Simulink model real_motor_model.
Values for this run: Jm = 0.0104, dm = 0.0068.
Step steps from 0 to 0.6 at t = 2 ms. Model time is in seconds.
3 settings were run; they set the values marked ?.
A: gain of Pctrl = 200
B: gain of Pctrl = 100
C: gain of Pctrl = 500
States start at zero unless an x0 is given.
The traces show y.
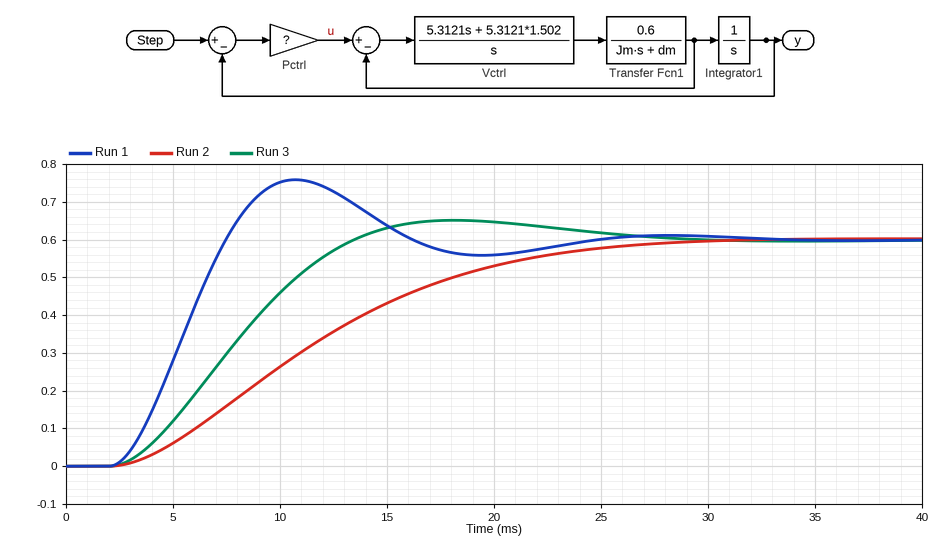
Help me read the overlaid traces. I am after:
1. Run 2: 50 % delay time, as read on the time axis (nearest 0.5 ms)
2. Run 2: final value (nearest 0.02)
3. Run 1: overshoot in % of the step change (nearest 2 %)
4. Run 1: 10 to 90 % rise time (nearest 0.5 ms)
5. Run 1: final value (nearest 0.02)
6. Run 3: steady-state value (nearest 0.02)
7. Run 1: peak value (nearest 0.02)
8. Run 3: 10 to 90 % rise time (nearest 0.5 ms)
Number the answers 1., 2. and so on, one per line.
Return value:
1. 11.0 ms
2. 0.60
3. 26 %
4. 3.5 ms
5. 0.60
6. 0.60
7. 0.76
8. 7.5 ms
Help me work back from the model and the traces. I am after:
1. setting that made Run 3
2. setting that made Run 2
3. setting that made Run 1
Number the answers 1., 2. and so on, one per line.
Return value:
1. A
2. B
3. C
